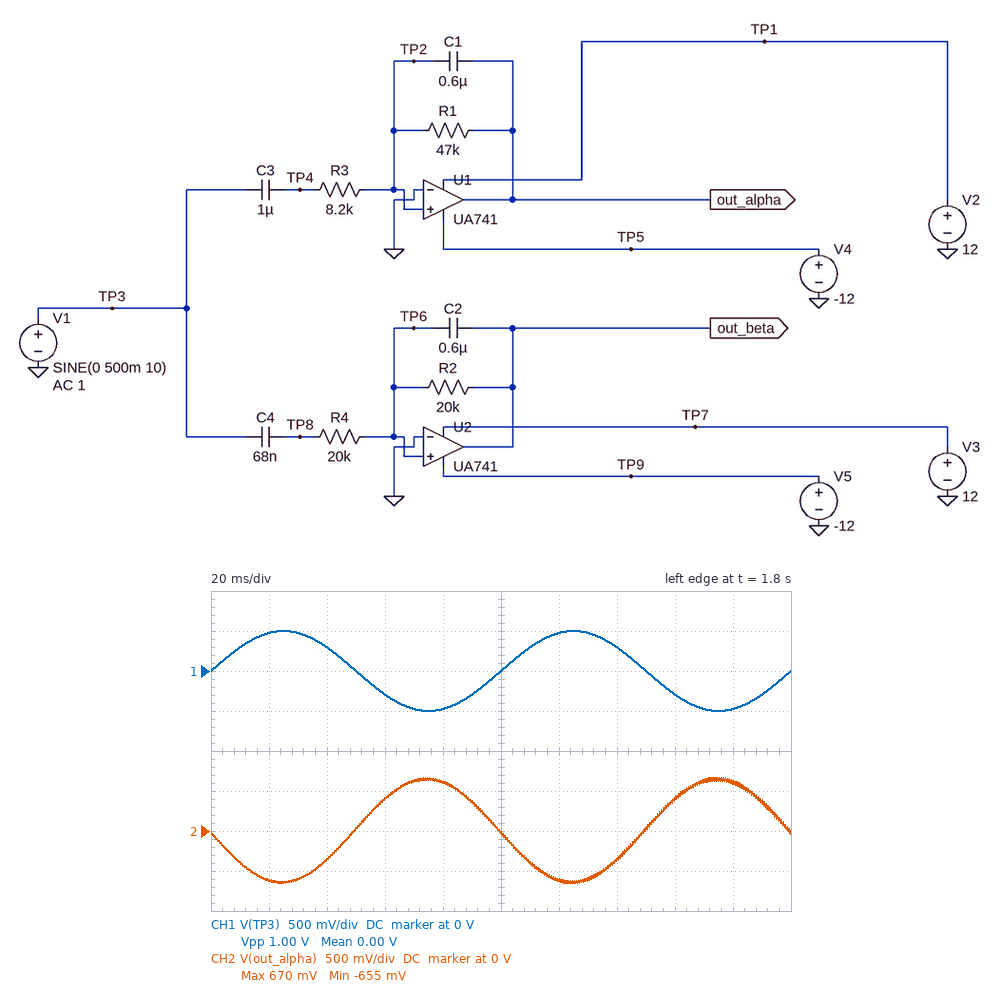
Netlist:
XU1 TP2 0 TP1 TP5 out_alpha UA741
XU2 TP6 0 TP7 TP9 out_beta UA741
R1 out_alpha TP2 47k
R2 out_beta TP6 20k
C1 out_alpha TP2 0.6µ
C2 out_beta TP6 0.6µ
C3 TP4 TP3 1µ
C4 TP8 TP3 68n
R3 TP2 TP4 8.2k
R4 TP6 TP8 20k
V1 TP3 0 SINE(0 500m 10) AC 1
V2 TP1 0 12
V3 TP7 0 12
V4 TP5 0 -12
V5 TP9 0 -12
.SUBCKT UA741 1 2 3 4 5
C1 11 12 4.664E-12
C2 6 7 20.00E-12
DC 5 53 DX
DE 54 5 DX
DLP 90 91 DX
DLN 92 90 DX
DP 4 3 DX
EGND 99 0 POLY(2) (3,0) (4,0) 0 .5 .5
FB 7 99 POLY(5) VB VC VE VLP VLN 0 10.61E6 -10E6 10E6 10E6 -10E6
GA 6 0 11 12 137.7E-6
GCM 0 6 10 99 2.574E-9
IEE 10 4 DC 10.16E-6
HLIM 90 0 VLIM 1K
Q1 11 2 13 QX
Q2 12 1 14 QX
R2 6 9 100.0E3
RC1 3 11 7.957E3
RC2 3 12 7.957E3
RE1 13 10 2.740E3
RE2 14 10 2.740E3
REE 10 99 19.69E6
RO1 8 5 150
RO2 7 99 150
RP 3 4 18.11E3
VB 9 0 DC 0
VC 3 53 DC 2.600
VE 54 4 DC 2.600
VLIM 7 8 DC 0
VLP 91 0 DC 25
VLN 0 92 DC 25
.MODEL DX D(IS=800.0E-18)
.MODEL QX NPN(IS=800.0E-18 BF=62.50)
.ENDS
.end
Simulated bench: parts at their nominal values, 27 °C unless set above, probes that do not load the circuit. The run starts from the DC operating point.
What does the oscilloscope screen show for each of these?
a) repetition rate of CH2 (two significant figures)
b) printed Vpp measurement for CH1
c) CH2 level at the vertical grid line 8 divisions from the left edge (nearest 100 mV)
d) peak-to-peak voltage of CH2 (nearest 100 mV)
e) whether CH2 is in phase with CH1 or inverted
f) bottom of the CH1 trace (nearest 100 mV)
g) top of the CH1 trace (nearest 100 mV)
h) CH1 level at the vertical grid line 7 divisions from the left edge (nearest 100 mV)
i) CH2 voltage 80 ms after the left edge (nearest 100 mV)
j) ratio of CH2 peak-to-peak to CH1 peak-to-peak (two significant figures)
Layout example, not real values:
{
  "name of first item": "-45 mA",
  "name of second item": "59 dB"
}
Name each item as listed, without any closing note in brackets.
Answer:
{
  "repetition rate of CH2": "10 Hz",
  "printed Vpp measurement for CH1": "1.00 V",
  "CH2 level at the vertical grid line 8 divisions from the left edge": "400 mV",
  "peak-to-peak voltage of CH2": "1.3 V",
  "whether CH2 is in phase with CH1 or inverted": "inverted",
  "bottom of the CH1 trace": "-500 mV",
  "top of the CH1 trace": "500 mV",
  "CH1 level at the vertical grid line 7 divisions from the left edge": "300 mV",
  "CH2 voltage 80 ms after the left edge": "600 mV",
  "ratio of CH2 peak-to-peak to CH1 peak-to-peak": "1.3"
}
